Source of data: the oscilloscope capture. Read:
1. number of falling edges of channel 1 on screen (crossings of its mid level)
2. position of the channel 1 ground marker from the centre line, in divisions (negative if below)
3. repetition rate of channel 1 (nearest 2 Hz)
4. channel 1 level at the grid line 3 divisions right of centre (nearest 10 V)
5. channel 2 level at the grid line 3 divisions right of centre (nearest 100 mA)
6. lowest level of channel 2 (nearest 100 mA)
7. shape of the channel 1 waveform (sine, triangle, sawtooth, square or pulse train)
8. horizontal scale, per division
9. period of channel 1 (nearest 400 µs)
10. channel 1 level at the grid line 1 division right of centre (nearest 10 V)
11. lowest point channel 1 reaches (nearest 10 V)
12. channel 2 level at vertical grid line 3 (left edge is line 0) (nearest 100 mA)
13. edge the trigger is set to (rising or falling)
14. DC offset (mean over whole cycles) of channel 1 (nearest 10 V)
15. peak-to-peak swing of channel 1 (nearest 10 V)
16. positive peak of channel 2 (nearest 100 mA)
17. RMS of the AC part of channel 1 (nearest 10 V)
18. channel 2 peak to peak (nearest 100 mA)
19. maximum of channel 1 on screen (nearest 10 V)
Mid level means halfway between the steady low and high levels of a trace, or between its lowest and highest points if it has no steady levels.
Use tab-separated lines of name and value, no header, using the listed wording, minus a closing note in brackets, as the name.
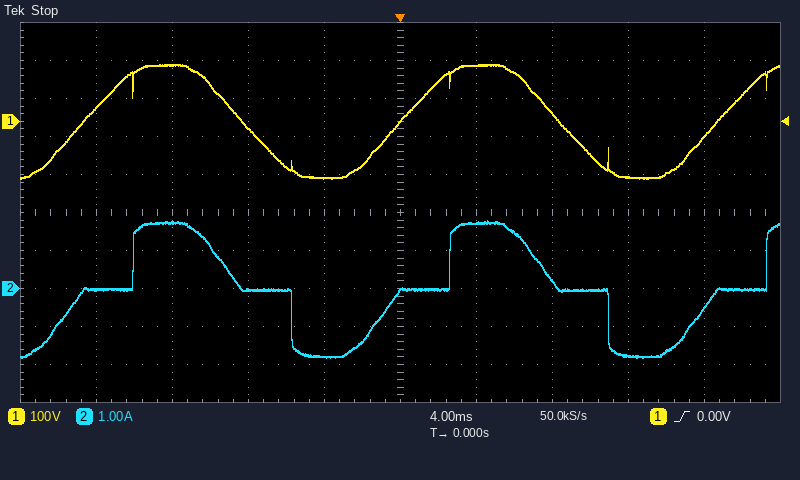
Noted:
number of falling edges of channel 1 on screen	2
position of the channel 1 ground marker from the centre line, in divisions	+2.4 div
repetition rate of channel 1	60 Hz
channel 1 level at the grid line 3 divisions right of centre	-150 V
channel 2 level at the grid line 3 divisions right of centre	-1.8 A
lowest level of channel 2	-1.8 A
shape of the channel 1 waveform	sine
horizontal scale, per division	4 ms
period of channel 1	16.8 ms
channel 1 level at the grid line 1 division right of centre	150 V
lowest point channel 1 reaches	-150 V
channel 2 level at vertical grid line 3 (left edge is line 0)	0.0 A
edge the trigger is set to	rising
DC offset (mean over whole cycles) of channel 1	0 V
peak-to-peak swing of channel 1	300 V
positive peak of channel 2	1.8 A
RMS of the AC part of channel 1	110 V
channel 2 peak to peak	3.6 A
maximum of channel 1 on screen	150 V
